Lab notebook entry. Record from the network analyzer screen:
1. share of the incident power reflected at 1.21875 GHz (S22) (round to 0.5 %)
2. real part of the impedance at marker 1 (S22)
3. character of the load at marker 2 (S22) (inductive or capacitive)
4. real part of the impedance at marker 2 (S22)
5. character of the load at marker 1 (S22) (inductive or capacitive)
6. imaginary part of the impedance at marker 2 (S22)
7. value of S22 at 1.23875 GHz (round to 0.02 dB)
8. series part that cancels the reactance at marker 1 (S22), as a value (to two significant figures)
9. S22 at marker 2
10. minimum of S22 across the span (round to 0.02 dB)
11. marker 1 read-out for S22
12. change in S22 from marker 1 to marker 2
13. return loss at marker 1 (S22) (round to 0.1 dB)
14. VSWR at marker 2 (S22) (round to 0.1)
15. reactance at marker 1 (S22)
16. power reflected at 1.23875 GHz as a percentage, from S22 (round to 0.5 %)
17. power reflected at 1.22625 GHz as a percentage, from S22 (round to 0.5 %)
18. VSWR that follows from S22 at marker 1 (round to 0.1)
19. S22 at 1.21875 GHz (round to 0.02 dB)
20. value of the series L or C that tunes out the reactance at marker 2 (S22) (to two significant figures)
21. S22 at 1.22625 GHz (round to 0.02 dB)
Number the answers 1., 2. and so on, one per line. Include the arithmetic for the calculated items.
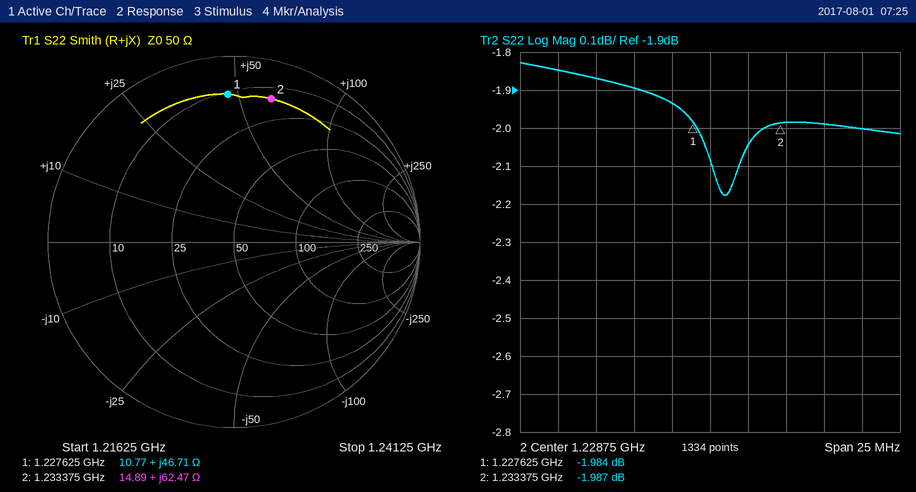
1. 10^(-1.84/10) ≈ 65.5 %
2. 10.77 Ω
3. inductive
4. 14.89 Ω
5. inductive
6. +62.47 Ω
7. -2.00 dB
8. C = 1/(2π × 1.227625 GHz × 46.71 Ω) ≈ 2.8 pF
9. -1.987 dB
10. -2.18 dB
11. -1.984 dB
12. -1.987 − (-1.984) = -0.003 dB
13. 2.0 dB
14. 8.8
15. +46.71 Ω
16. 10^(-2/10) ≈ 63.1 %, so 63.0 % to the nearest 0.5 %
17. 10^(-1.94/10) ≈ 64.0 %
18. (1 + 0.7958)/(1 − 0.7958) ≈ 8.8
19. -1.84 dB
20. C = 1/(2π × 1.233375 GHz × 62.47 Ω) ≈ 2.1 pF
21. -1.94 dB
